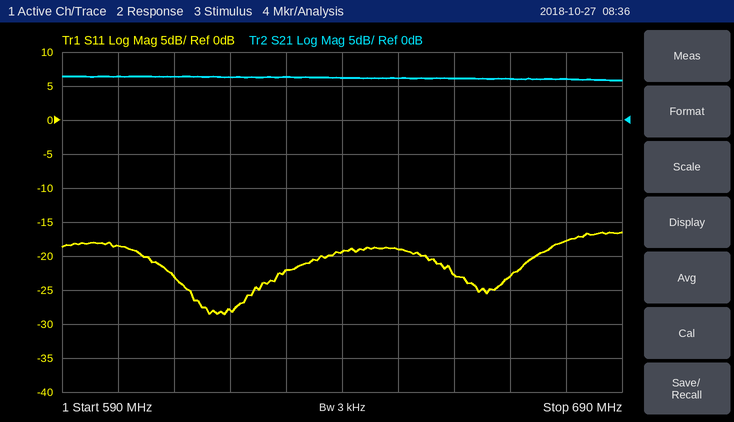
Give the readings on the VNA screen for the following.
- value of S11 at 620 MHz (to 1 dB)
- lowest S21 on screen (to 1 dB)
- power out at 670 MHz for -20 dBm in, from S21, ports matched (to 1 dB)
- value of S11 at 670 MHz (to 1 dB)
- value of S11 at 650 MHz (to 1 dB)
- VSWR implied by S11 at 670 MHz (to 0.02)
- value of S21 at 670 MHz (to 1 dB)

-28 dB
6 dB
-14 dBm
-23 dB
-19 dB
1.16
6 dB
